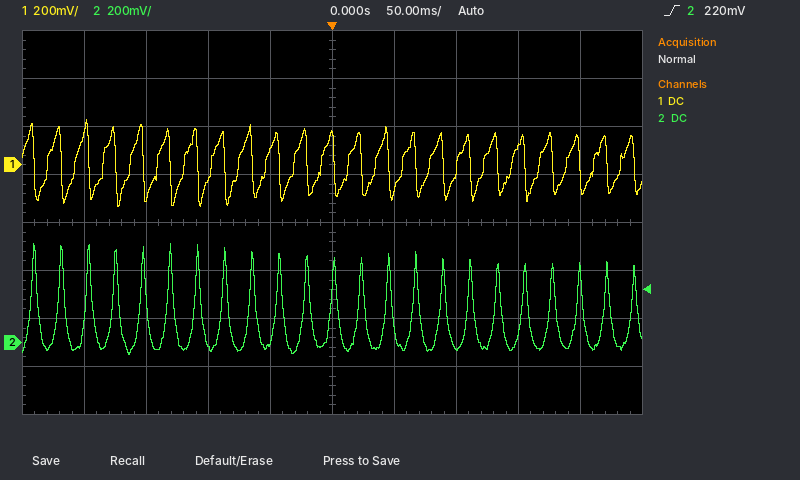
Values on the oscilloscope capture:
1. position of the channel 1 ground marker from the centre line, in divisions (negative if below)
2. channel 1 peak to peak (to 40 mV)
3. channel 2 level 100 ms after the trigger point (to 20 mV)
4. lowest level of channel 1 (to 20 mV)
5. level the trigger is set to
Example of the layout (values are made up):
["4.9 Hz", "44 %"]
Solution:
["+1.2 div", "360 mV", "-20 mV", "-180 mV", "220 mV"]
